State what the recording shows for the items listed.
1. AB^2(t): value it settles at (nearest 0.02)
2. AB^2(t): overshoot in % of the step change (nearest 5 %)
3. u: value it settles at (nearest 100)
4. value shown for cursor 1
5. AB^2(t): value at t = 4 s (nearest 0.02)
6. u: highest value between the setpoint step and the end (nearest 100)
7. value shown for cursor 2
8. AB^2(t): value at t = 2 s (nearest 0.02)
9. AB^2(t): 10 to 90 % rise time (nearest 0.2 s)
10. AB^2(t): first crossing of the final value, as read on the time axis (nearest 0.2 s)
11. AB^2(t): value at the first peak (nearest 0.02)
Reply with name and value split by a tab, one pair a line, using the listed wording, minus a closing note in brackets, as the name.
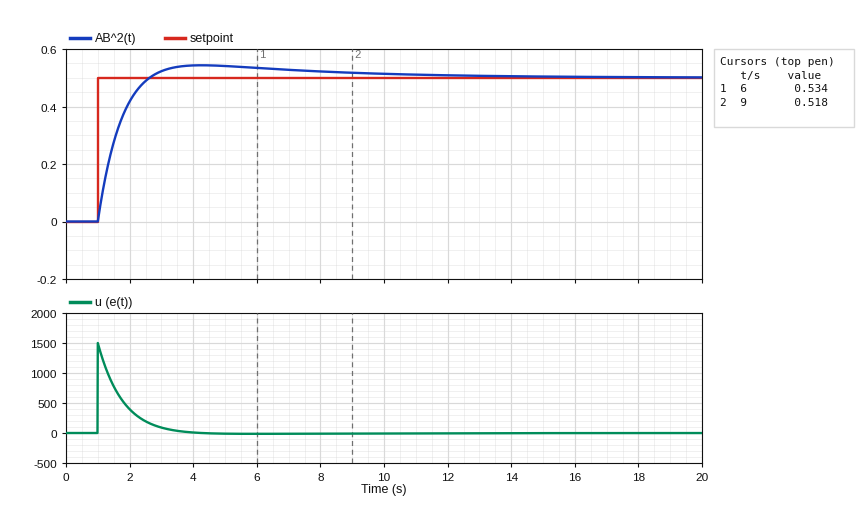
AB^2(t): value it settles at	0.50
AB^2(t): overshoot in % of the step change	10 %
u: value it settles at	0
value shown for cursor 1	0.534
AB^2(t): value at t = 4 s	0.54
u: highest value between the setpoint step and the end	1500
value shown for cursor 2	0.518
AB^2(t): value at t = 2 s	0.42
AB^2(t): 10 to 90 % rise time	1.2 s
AB^2(t): first crossing of the final value, as read on the time axis	2.6 s
AB^2(t): value at the first peak	0.54
